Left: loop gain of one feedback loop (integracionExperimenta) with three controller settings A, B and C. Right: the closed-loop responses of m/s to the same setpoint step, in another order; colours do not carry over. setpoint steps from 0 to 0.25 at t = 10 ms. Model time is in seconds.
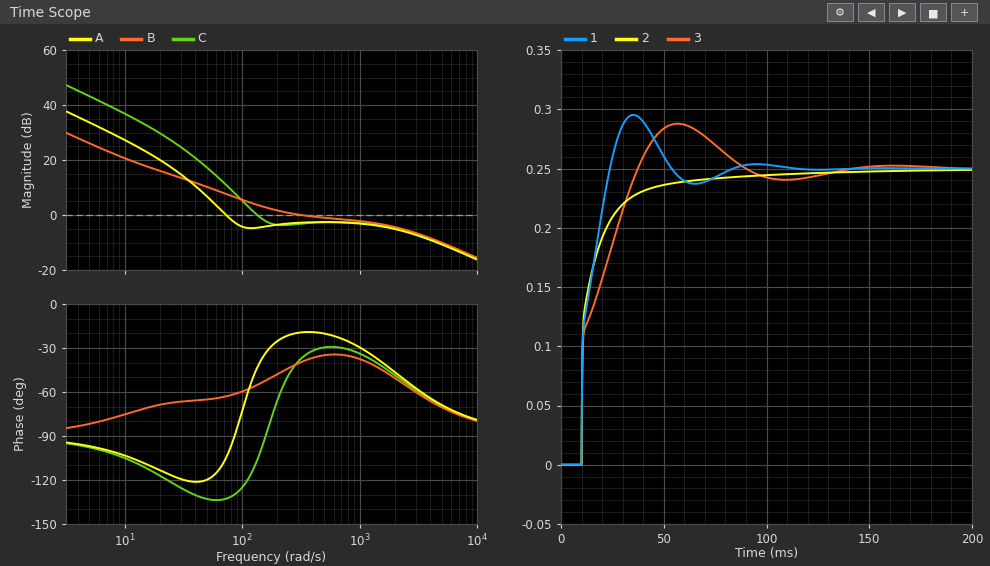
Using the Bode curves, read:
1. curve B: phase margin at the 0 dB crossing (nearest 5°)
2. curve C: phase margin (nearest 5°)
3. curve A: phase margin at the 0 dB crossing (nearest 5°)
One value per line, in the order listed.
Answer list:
140°
75°
75°
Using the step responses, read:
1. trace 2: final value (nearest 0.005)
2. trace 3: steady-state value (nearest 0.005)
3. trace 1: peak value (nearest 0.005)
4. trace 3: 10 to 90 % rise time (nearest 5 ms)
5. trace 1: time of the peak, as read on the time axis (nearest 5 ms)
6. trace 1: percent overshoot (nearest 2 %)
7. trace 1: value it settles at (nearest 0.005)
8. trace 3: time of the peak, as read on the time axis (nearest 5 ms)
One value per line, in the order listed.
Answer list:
0.250
0.250
0.295
20 ms
35 ms
18 %
0.250
55 ms
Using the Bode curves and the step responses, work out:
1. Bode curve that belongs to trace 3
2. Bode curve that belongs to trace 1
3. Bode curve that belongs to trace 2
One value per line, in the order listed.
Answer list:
A
C
B
